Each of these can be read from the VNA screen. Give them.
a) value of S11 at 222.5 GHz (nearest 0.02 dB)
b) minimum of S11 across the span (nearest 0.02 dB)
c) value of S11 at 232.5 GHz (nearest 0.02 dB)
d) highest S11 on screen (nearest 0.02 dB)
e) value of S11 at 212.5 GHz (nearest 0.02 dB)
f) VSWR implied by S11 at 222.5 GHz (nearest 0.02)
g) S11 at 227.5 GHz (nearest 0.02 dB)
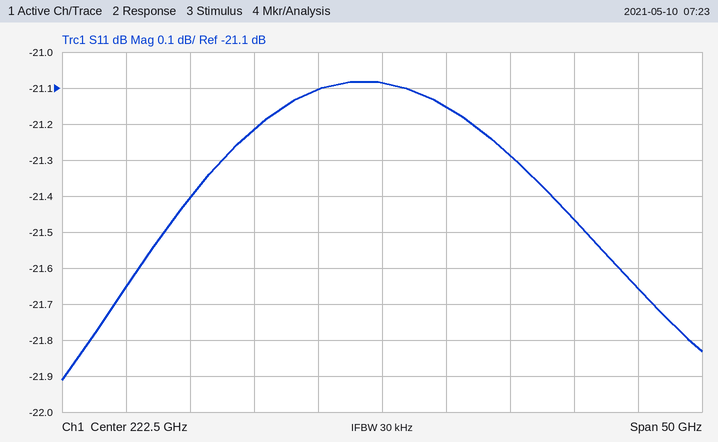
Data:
-21.08 dB
-21.92 dB
-21.28 dB
-21.08 dB
-21.22 dB
1.20
-21.16 dB
